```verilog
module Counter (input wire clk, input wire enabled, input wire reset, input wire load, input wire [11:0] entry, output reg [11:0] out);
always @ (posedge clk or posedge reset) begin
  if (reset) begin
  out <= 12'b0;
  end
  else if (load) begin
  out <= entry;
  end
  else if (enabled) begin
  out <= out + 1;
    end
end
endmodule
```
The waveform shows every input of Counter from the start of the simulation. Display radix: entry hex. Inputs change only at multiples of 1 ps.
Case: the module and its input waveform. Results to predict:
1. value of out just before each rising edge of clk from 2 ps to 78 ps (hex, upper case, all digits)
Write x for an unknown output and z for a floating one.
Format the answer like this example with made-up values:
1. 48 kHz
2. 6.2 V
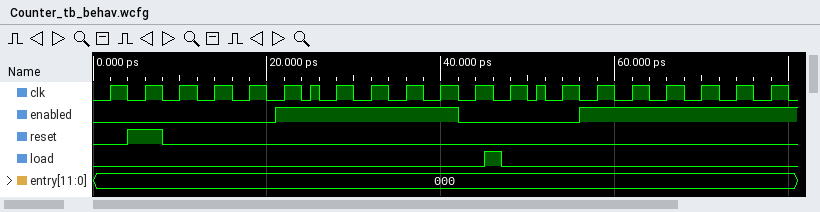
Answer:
1. x, 000, 000, 000, 000, 000, 001, 002, 003, 004, 005, 006, 006, 006, 006, 006, 007, 008, 009, 00A, 00B
